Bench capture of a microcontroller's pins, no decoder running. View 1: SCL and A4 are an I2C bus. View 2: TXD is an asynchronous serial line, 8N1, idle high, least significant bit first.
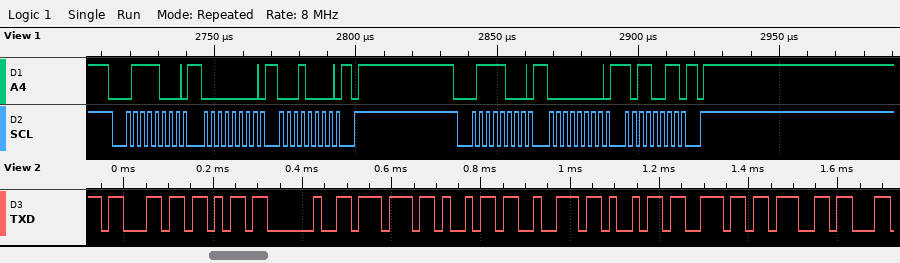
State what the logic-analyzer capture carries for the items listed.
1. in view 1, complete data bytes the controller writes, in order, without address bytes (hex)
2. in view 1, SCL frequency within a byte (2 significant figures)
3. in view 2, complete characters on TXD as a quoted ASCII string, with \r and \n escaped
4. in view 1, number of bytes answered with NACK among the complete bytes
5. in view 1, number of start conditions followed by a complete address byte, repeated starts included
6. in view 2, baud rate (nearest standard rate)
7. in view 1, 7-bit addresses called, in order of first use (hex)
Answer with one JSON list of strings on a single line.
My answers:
["00 10 00 B3", "400 kHz", "\"ck wiring\"", "0", "2", "57600 baud", "0x3C"]
